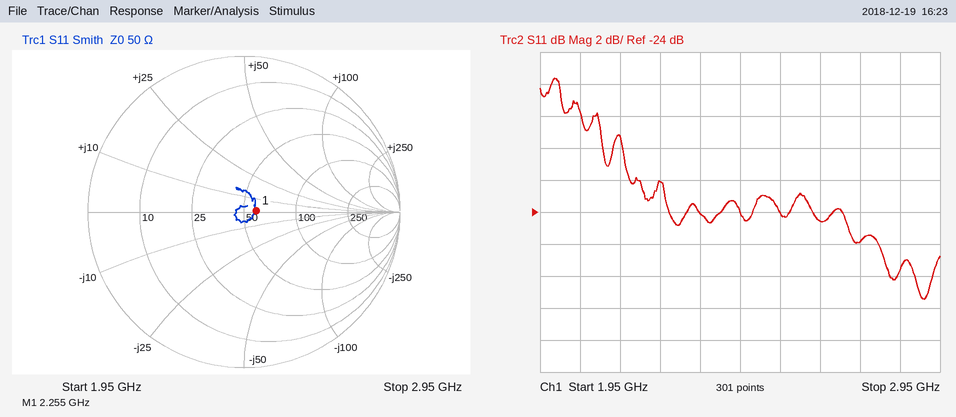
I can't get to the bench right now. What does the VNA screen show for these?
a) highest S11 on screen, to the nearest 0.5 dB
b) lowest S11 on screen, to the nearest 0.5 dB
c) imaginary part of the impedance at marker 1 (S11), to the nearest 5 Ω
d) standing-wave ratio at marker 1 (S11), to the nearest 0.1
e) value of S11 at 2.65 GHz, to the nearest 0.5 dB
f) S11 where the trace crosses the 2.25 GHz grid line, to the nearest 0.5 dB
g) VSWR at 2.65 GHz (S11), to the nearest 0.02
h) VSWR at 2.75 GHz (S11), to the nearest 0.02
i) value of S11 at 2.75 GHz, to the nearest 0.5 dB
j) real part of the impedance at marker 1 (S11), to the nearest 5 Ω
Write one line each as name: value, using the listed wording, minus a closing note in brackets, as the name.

highest S11 on screen, to the nearest 0.5 dB: -15.5 dB
lowest S11 on screen, to the nearest 0.5 dB: -29.5 dB
imaginary part of the impedance at marker 1 (S11), to the nearest 5 Ω: 0 Ω
standing-wave ratio at marker 1 (S11), to the nearest 0.1: 1.2
value of S11 at 2.65 GHz, to the nearest 0.5 dB: -24.5 dB
S11 where the trace crosses the 2.25 GHz grid line, to the nearest 0.5 dB: -22.0 dB
VSWR at 2.65 GHz (S11), to the nearest 0.02: 1.12
VSWR at 2.75 GHz (S11), to the nearest 0.02: 1.10
value of S11 at 2.75 GHz, to the nearest 0.5 dB: -26.0 dB
real part of the impedance at marker 1 (S11), to the nearest 5 Ω: 60 Ω
